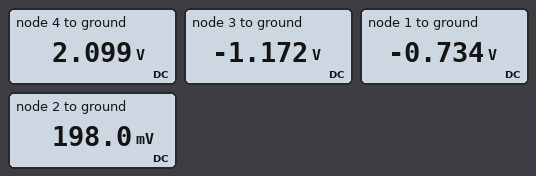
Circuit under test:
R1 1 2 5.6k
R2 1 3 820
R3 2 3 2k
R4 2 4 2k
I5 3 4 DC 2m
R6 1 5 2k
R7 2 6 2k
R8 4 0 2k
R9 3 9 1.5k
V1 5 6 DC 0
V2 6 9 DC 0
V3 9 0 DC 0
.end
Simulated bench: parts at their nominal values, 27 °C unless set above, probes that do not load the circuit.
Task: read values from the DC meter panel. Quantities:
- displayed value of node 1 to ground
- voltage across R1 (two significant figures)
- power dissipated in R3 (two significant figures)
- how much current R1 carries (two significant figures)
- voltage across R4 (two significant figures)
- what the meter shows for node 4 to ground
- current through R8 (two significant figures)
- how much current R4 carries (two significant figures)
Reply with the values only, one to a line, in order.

-0.734 V
930 mV
940 µW
170 µA
1.9 V
2.099 V
1.0 mA
950 µA
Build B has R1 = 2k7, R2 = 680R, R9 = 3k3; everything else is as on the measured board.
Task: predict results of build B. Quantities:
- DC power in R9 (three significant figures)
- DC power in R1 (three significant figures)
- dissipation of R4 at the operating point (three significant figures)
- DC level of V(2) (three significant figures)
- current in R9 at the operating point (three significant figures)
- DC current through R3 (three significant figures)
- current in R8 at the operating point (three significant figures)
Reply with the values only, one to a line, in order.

702 µW
296 µW
2.07 mW
-73.5 mV
461 µA
724 µA
982 µA
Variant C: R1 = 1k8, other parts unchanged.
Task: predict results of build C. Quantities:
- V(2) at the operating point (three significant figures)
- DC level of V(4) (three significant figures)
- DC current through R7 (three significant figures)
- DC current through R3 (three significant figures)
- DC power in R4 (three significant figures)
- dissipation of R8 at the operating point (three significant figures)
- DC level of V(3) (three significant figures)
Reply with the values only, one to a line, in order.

60.7 mV
2.03 V
30.3 µA
594 µA
1.94 mW
2.06 mW
-1.13 V
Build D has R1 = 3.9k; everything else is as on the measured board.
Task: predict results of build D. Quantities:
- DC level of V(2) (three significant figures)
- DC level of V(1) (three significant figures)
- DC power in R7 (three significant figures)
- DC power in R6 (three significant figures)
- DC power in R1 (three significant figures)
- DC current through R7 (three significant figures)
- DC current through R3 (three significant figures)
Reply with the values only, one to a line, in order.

161 mV
-695 mV
12.9 µW
241 µW
188 µW
80.3 µA
660 µA
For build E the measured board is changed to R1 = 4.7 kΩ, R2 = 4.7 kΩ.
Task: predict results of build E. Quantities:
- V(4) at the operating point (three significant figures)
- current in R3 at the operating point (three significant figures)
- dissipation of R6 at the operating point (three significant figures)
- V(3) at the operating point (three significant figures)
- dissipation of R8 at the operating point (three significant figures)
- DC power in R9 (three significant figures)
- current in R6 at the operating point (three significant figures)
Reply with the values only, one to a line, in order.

2.07 V
795 µA
44.3 µW
-1.44 V
2.15 mW
1.39 mW
149 µA
